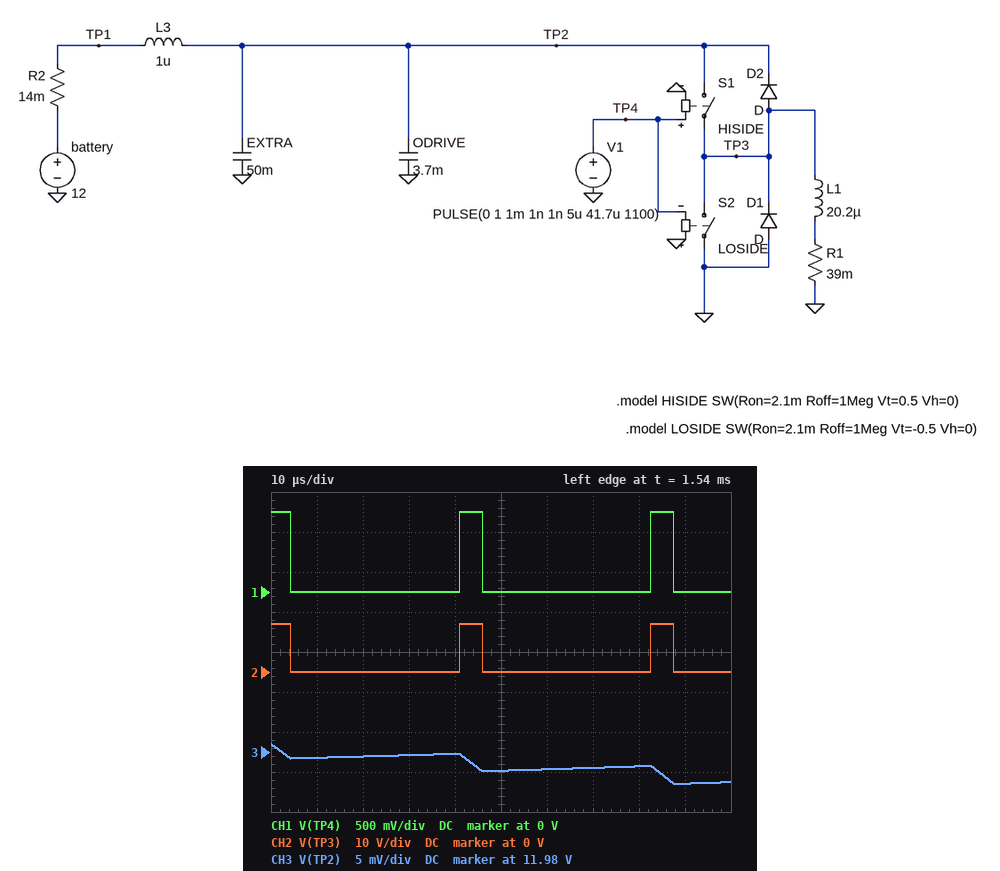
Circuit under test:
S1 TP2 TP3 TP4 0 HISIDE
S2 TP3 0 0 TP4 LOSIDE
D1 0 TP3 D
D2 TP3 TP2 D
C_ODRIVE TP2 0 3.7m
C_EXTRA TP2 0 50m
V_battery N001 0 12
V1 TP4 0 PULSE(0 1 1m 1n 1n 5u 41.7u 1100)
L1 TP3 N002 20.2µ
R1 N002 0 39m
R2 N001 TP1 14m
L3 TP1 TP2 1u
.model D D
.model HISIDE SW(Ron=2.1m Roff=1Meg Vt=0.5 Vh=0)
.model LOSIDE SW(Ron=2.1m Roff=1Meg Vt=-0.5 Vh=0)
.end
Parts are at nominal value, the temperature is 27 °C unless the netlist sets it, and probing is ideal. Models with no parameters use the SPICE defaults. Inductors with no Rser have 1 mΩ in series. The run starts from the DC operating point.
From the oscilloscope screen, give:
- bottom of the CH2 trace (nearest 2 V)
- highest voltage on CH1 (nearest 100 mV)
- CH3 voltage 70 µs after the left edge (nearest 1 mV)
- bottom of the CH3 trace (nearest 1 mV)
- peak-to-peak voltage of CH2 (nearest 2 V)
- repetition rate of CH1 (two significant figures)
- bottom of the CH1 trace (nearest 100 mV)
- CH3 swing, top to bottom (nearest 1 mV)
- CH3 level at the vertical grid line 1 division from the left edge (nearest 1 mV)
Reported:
0 V
1.0 V
11.983 V
11.981 V
12 V
24 kHz
0 V
5 mV
11.984 V
